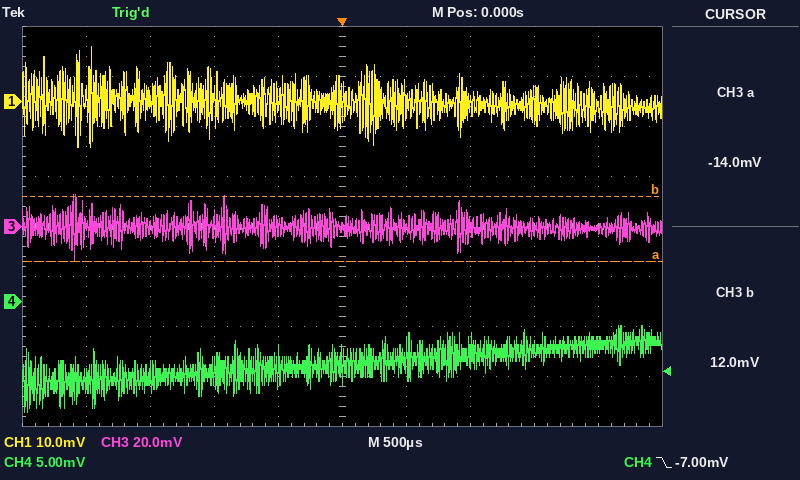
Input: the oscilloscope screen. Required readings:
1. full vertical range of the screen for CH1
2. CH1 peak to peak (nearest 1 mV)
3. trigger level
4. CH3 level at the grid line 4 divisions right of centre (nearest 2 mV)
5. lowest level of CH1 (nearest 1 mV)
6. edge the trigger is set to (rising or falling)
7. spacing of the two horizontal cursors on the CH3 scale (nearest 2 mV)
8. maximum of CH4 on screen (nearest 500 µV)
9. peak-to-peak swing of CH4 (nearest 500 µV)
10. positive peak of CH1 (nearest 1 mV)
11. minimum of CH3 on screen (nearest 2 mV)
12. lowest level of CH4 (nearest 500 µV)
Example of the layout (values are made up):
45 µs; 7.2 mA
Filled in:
80 mV; 20 mV; -7.00 mV; 0 mV; -9 mV; falling; 26 mV; -2.5 mV; 8.5 mV; 11 mV; -14 mV; -11.0 mV
